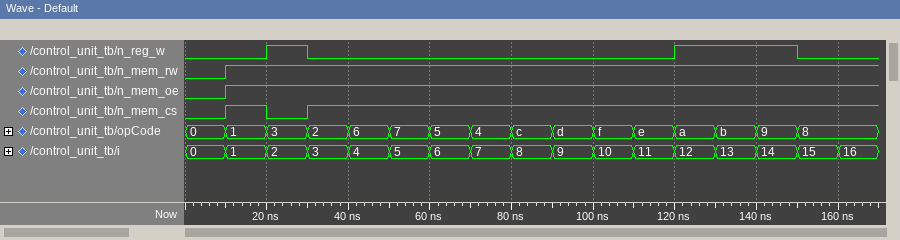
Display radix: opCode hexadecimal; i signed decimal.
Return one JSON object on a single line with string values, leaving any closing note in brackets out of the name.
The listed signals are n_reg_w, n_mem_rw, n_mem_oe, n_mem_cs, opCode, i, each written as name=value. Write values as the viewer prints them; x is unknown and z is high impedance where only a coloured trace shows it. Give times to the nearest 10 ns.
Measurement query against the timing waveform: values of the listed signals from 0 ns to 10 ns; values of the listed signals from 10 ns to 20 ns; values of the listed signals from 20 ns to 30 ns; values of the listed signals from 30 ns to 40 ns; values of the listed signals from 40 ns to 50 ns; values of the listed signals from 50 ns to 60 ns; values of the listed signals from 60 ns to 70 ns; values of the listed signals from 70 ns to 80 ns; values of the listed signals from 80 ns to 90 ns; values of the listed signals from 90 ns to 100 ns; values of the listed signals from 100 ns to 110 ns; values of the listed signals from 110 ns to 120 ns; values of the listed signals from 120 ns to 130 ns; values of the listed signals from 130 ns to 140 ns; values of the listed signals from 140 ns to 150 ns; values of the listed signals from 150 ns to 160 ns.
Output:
{"values of the listed signals from 0 ns to 10 ns": "n_reg_w=0, n_mem_rw=0, n_mem_oe=0, n_mem_cs=0, opCode=0, i=0", "values of the listed signals from 10 ns to 20 ns": "n_reg_w=0, n_mem_rw=1, n_mem_oe=1, n_mem_cs=1, opCode=1, i=1", "values of the listed signals from 20 ns to 30 ns": "n_reg_w=1, n_mem_rw=1, n_mem_oe=1, n_mem_cs=0, opCode=3, i=2", "values of the listed signals from 30 ns to 40 ns": "n_reg_w=0, n_mem_rw=1, n_mem_oe=1, n_mem_cs=1, opCode=2, i=3", "values of the listed signals from 40 ns to 50 ns": "n_reg_w=0, n_mem_rw=1, n_mem_oe=1, n_mem_cs=1, opCode=6, i=4", "values of the listed signals from 50 ns to 60 ns": "n_reg_w=0, n_mem_rw=1, n_mem_oe=1, n_mem_cs=1, opCode=7, i=5", "values of the listed signals from 60 ns to 70 ns": "n_reg_w=0, n_mem_rw=1, n_mem_oe=1, n_mem_cs=1, opCode=5, i=6", "values of the listed signals from 70 ns to 80 ns": "n_reg_w=0, n_mem_rw=1, n_mem_oe=1, n_mem_cs=1, opCode=4, i=7", "values of the listed signals from 80 ns to 90 ns": "n_reg_w=0, n_mem_rw=1, n_mem_oe=1, n_mem_cs=1, opCode=c, i=8", "values of the listed signals from 90 ns to 100 ns": "n_reg_w=0, n_mem_rw=1, n_mem_oe=1, n_mem_cs=1, opCode=d, i=9", "values of the listed signals from 100 ns to 110 ns": "n_reg_w=0, n_mem_rw=1, n_mem_oe=1, n_mem_cs=1, opCode=f, i=10", "values of the listed signals from 110 ns to 120 ns": "n_reg_w=0, n_mem_rw=1, n_mem_oe=1, n_mem_cs=1, opCode=e, i=11", "values of the listed signals from 120 ns to 130 ns": "n_reg_w=1, n_mem_rw=1, n_mem_oe=1, n_mem_cs=1, opCode=a, i=12", "values of the listed signals from 130 ns to 140 ns": "n_reg_w=1, n_mem_rw=1, n_mem_oe=1, n_mem_cs=1, opCode=b, i=13", "values of the listed signals from 140 ns to 150 ns": "n_reg_w=1, n_mem_rw=1, n_mem_oe=1, n_mem_cs=1, opCode=9, i=14", "values of the listed signals from 150 ns to 160 ns": "n_reg_w=0, n_mem_rw=1, n_mem_oe=1, n_mem_cs=1, opCode=8, i=15"}
